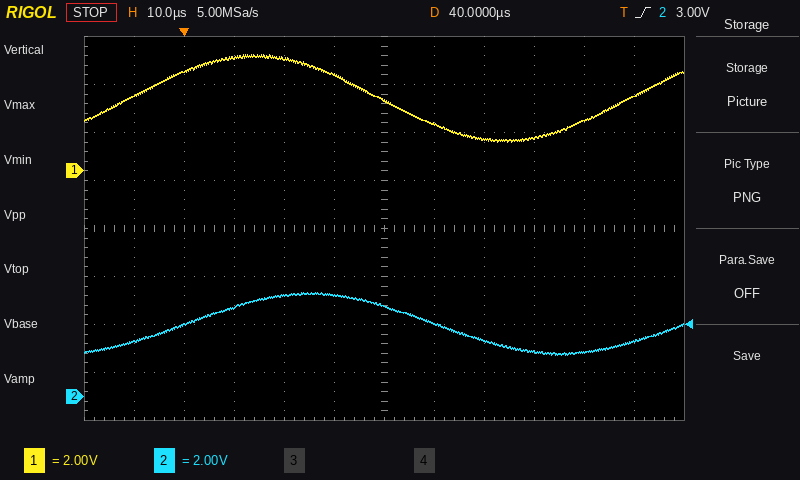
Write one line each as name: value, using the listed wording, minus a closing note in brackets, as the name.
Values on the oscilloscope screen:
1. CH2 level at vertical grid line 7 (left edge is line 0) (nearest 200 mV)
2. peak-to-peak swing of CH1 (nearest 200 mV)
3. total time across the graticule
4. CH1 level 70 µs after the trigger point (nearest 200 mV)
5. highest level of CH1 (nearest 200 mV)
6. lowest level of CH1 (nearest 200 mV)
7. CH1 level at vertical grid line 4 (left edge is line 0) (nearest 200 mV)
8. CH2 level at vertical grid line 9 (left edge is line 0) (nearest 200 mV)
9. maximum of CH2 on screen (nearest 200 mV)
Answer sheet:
CH2 level at vertical grid line 7 (left edge is line 0): 3.0 V
peak-to-peak swing of CH1: 3.6 V
total time across the graticule: 120 µs
CH1 level 70 µs after the trigger point: 1.4 V
highest level of CH1: 4.8 V
lowest level of CH1: 1.2 V
CH1 level at vertical grid line 4 (left edge is line 0): 4.6 V
CH2 level at vertical grid line 9 (left edge is line 0): 1.8 V
maximum of CH2 on screen: 4.4 V
